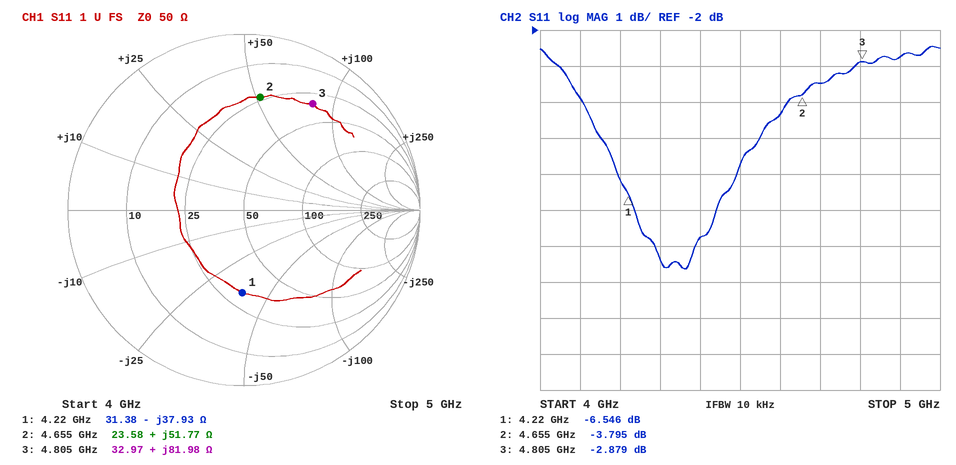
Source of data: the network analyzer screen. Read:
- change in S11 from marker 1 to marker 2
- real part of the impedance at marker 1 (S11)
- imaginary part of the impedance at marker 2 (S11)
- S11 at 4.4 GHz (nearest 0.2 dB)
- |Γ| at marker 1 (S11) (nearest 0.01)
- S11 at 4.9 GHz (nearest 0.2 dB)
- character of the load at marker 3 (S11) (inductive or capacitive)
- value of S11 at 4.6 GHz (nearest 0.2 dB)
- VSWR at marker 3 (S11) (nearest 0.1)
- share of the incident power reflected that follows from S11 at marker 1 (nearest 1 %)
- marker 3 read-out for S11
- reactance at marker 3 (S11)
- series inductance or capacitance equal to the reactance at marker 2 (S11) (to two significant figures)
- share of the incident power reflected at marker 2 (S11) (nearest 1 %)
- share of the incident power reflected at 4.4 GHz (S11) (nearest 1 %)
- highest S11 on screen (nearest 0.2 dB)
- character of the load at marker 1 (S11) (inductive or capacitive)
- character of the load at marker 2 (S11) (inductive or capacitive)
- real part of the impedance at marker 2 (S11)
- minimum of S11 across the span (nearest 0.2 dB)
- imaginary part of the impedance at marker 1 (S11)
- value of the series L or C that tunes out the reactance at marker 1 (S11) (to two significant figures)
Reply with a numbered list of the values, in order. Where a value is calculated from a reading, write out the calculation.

1. -3.795 − (-6.546) = 2.751 dB
2. 31.38 Ω
3. +51.77 Ω
4. -7.8 dB
5. 0.47
6. -2.8 dB
7. inductive
8. -4.4 dB
9. 6.1
10. 10^(-6.546/10) ≈ 22 %
11. -2.879 dB
12. +81.98 Ω
13. L = 51.77 Ω/(2π × 4.655 GHz) ≈ 1.8 nH
14. 10^(-3.795/10) ≈ 42 %
15. 10^(-7.8/10) ≈ 17 %
16. -2.4 dB
17. capacitive
18. inductive
19. 23.58 Ω
20. -8.6 dB
21. -37.93 Ω
22. L = 37.93 Ω/(2π × 4.22 GHz) ≈ 1.4 nH
